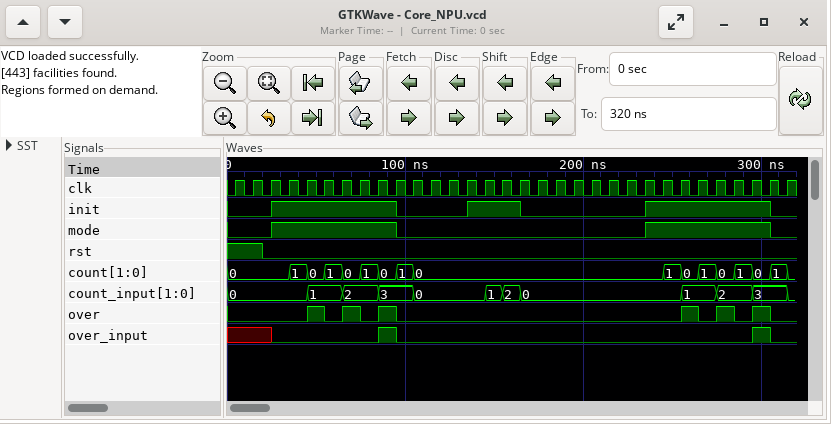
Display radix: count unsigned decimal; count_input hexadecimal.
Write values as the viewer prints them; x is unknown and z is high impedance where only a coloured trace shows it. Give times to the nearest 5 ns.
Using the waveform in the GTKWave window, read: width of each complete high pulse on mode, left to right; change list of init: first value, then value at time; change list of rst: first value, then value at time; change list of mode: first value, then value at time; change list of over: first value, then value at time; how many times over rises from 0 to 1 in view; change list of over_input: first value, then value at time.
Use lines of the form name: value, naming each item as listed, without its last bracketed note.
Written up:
width of each complete high pulse on mode, left to right: 70 ns, 70 ns
change list of init: first value, then value at time: 0, 1 at 25 ns, 0 at 95 ns, 1 at 135 ns, 0 at 165 ns, 1 at 235 ns, 0 at 305 ns
change list of rst: first value, then value at time: 1, 0 at 20 ns
change list of mode: first value, then value at time: 0, 1 at 25 ns, 0 at 95 ns, 1 at 235 ns, 0 at 305 ns
change list of over: first value, then value at time: 0, 1 at 45 ns, 0 at 55 ns, 1 at 65 ns, 0 at 75 ns, 1 at 85 ns, 0 at 95 ns, 1 at 255 ns, 0 at 265 ns, 1 at 275 ns, 0 at 285 ns, 1 at 295 ns, 0 at 305 ns
how many times over rises from 0 to 1 in view: 6
change list of over_input: first value, then value at time: x, 0 at 25 ns, 1 at 85 ns, 0 at 95 ns, 1 at 295 ns, 0 at 305 ns
